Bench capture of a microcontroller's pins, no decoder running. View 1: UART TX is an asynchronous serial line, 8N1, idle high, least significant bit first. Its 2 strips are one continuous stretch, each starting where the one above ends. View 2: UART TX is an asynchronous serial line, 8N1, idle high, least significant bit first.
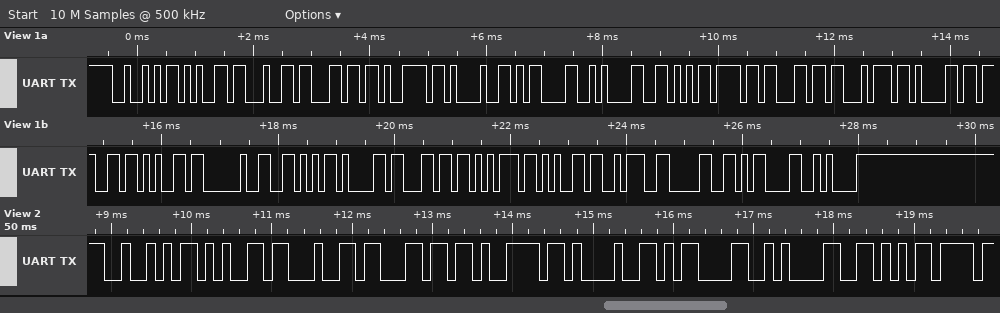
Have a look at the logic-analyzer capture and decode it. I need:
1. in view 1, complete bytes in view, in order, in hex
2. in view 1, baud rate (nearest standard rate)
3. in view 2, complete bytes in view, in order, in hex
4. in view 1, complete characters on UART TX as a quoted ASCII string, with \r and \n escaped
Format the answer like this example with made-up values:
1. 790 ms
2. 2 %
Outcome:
1. 52 65 64 6C 79 21 0D 0A 56 6F 6C 74 61 67 65 20 56 61 6C 75 65 3A 30 0D 0A
2. 9600 baud
3. 52 65 64 6C 79 21 0D 0A 56
4. "Redly!\r\nVoltage Value:0\r\n"
